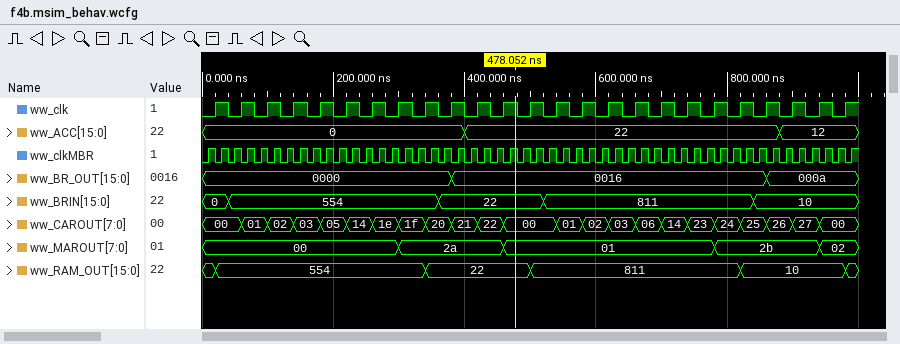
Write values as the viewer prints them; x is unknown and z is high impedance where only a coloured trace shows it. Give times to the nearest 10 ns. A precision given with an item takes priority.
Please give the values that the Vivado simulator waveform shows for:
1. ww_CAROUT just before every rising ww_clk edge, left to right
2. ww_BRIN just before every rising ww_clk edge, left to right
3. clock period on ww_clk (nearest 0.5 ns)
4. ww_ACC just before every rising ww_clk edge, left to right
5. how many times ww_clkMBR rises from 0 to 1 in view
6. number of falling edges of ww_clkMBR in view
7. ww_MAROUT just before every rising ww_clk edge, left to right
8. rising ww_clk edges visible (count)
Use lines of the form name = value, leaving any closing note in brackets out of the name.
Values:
ww_CAROUT just before every rising ww_clk edge, left to right = 00, 00, 01, 02, 03, 05, 14, 1e, 1f, 20, 21, 22, 00, 00, 01, 02, 03, 06, 14, 23, 24, 25, 26, 27, 00
ww_BRIN just before every rising ww_clk edge, left to right = 0, 554, 554, 554, 554, 554, 554, 554, 554, 22, 22, 22, 22, 811, 811, 811, 811, 811, 811, 811, 811, 10, 10, 10, 10
clock period on ww_clk = 40 ns
ww_ACC just before every rising ww_clk edge, left to right = 0, 0, 0, 0, 0, 0, 0, 0, 0, 0, 22, 22, 22, 22, 22, 22, 22, 22, 22, 22, 22, 22, 12, 12, 12
how many times ww_clkMBR rises from 0 to 1 in view = 50
number of falling edges of ww_clkMBR in view = 49
ww_MAROUT just before every rising ww_clk edge, left to right = 00, 00, 00, 00, 00, 00, 00, 00, 2a, 2a, 2a, 2a, 01, 01, 01, 01, 01, 01, 01, 01, 2b, 2b, 2b, 2b, 02
rising ww_clk edges visible = 25
